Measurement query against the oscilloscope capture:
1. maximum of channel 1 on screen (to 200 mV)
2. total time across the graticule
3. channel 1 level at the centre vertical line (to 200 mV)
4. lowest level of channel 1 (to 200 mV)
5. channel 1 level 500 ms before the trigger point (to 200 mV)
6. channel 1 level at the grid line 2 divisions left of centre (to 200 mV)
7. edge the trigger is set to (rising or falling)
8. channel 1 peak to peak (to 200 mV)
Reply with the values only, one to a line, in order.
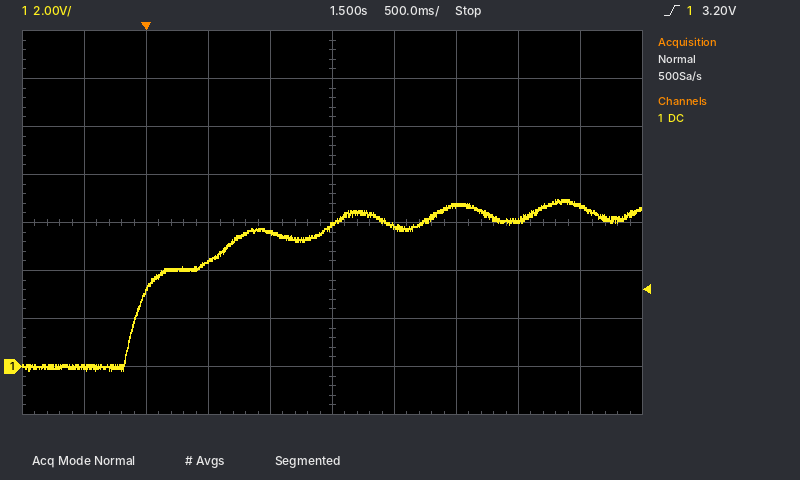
7.0 V
5 s
5.8 V
-200 mV
0.0 V
4.4 V
rising
7.2 V
